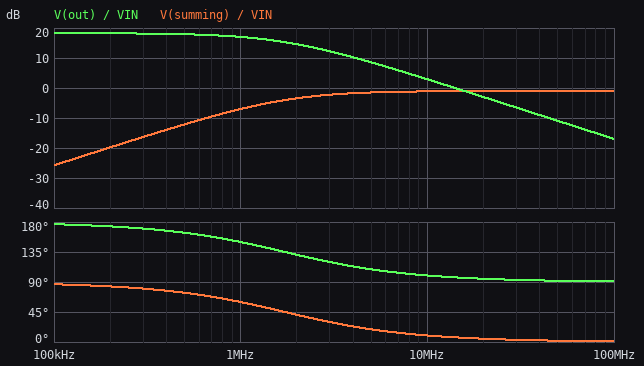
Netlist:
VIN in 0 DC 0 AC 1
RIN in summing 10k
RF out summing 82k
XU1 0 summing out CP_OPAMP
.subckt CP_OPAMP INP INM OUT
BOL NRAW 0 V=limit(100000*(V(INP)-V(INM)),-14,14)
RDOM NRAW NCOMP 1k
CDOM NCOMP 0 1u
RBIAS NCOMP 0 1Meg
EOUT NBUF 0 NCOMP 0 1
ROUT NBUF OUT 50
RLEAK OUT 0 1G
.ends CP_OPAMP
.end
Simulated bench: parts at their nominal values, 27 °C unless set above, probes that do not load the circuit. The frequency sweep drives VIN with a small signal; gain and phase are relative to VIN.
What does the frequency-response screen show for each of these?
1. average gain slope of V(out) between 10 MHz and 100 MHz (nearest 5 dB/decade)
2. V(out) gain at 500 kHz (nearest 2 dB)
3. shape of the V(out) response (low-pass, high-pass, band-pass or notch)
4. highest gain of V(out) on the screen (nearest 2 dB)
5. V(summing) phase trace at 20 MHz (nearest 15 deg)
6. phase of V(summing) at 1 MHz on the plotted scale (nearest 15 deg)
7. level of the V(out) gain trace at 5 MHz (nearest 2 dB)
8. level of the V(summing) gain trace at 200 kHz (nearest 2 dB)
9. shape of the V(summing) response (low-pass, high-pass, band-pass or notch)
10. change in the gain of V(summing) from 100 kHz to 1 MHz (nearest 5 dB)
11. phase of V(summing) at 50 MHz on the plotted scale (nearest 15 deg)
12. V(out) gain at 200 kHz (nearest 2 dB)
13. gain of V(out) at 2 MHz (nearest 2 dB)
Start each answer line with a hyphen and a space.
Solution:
- -20 dB/decade
- 18 dB
- low-pass
- 18 dB
- 0 deg
- 60 deg
- 8 dB
- -20 dB
- high-pass
- 20 dB
- 0 deg
- 18 dB
- 14 dB
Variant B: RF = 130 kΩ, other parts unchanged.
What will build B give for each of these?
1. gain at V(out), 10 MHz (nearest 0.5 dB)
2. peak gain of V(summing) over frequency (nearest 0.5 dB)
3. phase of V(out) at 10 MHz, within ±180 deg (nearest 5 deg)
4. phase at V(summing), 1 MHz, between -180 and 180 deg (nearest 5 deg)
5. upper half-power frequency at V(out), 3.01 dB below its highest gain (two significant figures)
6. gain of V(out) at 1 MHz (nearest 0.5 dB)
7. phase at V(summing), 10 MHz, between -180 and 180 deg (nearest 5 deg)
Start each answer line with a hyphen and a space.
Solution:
- 3.5 dB
- -0.5 dB
- 95 deg
- 50 deg
- 1.1 MHz
- 20.0 dB
- 5 deg
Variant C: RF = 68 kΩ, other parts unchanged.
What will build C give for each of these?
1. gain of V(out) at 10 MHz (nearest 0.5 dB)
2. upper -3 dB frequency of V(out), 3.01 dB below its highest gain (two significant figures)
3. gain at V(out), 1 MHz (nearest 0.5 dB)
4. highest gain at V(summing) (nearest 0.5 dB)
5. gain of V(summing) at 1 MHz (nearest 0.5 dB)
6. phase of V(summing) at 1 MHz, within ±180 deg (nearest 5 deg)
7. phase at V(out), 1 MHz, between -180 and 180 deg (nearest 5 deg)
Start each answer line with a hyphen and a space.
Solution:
- 2.5 dB
- 2.0 MHz
- 15.5 dB
- -1.0 dB
- -8.5 dB
- 65 deg
- 155 deg
